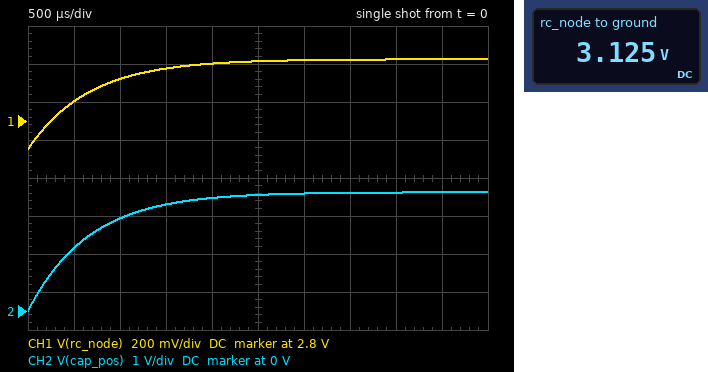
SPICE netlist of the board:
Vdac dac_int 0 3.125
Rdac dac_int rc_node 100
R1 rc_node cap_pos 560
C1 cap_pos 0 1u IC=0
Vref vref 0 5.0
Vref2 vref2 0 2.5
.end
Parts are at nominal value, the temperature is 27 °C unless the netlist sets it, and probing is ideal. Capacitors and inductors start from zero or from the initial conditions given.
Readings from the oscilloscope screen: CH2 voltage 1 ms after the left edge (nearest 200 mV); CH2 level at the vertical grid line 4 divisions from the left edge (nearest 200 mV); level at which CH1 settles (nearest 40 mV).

2.4 V
3.0 V
3.12 V
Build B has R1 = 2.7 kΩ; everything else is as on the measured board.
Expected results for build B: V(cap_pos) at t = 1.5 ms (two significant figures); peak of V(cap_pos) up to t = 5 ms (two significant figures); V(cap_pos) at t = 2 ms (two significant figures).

1.3 V
2.6 V
1.6 V
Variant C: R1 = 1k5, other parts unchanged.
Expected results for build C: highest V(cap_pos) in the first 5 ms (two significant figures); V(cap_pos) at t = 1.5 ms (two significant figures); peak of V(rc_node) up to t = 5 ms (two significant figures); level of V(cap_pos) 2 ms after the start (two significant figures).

3.0 V
1.9 V
3.1 V
2.2 V
